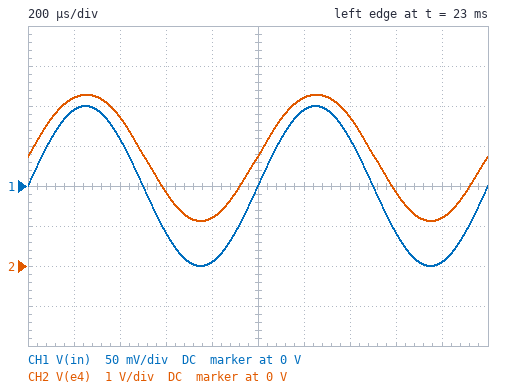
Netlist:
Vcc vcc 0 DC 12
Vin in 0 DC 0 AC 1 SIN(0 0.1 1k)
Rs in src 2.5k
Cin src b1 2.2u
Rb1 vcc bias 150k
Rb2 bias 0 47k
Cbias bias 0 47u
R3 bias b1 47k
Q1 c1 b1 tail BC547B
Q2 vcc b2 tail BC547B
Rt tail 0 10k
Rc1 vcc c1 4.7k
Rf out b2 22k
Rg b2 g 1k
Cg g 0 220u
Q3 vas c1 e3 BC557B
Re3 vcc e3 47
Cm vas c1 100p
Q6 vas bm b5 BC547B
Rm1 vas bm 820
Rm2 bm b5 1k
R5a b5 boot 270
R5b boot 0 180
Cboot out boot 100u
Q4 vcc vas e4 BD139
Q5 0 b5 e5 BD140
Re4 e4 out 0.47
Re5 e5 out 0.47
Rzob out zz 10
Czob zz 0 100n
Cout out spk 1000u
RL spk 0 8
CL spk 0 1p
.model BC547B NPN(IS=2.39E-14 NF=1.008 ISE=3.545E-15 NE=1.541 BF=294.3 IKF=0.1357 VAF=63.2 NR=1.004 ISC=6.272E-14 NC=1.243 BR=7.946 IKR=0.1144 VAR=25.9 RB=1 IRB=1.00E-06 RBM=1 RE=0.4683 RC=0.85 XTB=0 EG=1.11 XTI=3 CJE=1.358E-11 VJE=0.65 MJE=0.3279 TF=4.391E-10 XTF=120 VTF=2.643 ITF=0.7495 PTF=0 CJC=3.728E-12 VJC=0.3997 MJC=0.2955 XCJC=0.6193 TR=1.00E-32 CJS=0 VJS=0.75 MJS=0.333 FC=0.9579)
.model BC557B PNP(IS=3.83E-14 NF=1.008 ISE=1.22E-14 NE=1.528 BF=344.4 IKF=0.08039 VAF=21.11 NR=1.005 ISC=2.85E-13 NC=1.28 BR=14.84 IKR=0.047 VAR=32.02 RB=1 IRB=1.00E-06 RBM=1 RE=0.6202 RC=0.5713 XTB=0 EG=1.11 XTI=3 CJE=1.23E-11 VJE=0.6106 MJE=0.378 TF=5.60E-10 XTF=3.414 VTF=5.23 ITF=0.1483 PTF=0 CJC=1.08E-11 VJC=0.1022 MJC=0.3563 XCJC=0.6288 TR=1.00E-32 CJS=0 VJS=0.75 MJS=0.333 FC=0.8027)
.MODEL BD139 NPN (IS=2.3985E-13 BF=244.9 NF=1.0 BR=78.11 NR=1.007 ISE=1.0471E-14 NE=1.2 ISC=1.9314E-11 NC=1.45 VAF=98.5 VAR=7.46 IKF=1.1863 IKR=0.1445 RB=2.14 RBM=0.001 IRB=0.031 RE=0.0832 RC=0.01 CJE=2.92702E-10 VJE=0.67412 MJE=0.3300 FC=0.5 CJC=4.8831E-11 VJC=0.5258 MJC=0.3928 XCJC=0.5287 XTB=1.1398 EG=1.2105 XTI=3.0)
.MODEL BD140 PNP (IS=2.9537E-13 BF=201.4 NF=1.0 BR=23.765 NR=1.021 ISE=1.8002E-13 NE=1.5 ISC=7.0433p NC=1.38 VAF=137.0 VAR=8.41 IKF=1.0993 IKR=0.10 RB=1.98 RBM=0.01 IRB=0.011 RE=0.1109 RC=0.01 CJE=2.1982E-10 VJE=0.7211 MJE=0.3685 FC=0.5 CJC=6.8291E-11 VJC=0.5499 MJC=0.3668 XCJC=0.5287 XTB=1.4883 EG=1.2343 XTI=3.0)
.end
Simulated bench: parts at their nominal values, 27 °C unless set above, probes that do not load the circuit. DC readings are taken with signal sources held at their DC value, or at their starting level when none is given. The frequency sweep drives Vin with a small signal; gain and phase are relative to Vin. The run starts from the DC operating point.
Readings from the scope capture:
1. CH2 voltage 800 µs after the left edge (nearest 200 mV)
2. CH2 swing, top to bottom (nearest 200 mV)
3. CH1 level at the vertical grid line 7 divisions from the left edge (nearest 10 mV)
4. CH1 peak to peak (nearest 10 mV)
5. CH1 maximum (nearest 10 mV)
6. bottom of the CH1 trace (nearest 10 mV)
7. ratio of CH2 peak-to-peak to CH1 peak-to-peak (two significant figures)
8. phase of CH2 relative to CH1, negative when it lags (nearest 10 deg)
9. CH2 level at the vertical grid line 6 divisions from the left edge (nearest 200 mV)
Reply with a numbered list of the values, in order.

1. 1.2 V
2. 3.2 V
3. 60 mV
4. 200 mV
5. 100 mV
6. -100 mV
7. 16
8. 0 deg
9. 4.2 V
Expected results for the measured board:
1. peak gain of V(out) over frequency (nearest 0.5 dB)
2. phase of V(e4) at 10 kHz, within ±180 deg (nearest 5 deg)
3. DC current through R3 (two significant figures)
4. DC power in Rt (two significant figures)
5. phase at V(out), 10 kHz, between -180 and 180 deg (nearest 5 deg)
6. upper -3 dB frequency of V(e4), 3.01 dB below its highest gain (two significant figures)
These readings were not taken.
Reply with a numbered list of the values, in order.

1. 23.5 dB
2. -10 deg
3. 620 nA
4. 490 µW
5. -10 deg
6. 49 kHz
